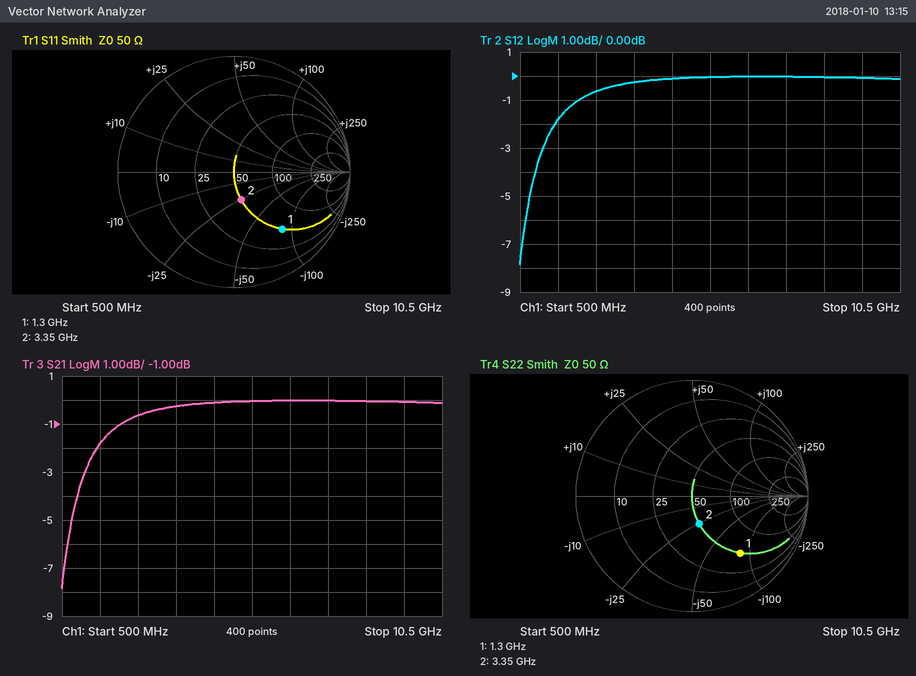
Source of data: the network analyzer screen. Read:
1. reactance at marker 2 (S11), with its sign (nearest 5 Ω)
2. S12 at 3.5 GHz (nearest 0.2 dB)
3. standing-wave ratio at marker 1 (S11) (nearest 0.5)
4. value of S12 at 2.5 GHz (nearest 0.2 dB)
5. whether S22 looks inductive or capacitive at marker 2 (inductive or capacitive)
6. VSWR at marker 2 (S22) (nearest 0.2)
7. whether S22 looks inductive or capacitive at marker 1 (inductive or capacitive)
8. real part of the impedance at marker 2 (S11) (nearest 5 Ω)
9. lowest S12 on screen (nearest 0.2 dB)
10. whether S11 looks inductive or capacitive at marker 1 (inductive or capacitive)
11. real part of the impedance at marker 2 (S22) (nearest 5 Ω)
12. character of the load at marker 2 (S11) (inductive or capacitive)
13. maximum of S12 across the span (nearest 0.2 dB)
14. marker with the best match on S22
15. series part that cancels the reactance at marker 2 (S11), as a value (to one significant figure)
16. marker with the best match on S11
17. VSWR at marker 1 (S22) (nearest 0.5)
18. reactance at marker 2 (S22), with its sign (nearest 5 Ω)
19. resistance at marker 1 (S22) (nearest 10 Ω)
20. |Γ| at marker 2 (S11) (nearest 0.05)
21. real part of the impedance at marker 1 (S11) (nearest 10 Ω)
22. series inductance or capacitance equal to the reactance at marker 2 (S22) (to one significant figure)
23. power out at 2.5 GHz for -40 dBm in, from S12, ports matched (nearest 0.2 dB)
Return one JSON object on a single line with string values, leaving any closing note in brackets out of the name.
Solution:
{"reactance at marker 2 (S11), with its sign": "-25 Ω", "S12 at 3.5 GHz": "-0.2 dB", "standing-wave ratio at marker 1 (S11)": "4.5", "value of S12 at 2.5 GHz": "-0.6 dB", "whether S22 looks inductive or capacitive at marker 2": "capacitive", "VSWR at marker 2 (S22)": "1.6", "whether S22 looks inductive or capacitive at marker 1": "capacitive", "real part of the impedance at marker 2 (S11)": "50 Ω", "lowest S12 on screen": "-7.8 dB", "whether S11 looks inductive or capacitive at marker 1": "capacitive", "real part of the impedance at marker 2 (S22)": "50 Ω", "character of the load at marker 2 (S11)": "capacitive", "maximum of S12 across the span": "0.0 dB", "marker with the best match on S22": "marker 2", "series part that cancels the reactance at marker 2 (S11), as a value": "1 nH", "marker with the best match on S11": "marker 2", "VSWR at marker 1 (S22)": "4.5", "reactance at marker 2 (S22), with its sign": "-25 Ω", "resistance at marker 1 (S22)": "50 Ω", "|Γ| at marker 2 (S11)": "0.25", "real part of the impedance at marker 1 (S11)": "50 Ω", "series inductance or capacitance equal to the reactance at marker 2 (S22)": "2 pF", "power out at 2.5 GHz for -40 dBm in, from S12, ports matched": "-40.6 dBm"}
